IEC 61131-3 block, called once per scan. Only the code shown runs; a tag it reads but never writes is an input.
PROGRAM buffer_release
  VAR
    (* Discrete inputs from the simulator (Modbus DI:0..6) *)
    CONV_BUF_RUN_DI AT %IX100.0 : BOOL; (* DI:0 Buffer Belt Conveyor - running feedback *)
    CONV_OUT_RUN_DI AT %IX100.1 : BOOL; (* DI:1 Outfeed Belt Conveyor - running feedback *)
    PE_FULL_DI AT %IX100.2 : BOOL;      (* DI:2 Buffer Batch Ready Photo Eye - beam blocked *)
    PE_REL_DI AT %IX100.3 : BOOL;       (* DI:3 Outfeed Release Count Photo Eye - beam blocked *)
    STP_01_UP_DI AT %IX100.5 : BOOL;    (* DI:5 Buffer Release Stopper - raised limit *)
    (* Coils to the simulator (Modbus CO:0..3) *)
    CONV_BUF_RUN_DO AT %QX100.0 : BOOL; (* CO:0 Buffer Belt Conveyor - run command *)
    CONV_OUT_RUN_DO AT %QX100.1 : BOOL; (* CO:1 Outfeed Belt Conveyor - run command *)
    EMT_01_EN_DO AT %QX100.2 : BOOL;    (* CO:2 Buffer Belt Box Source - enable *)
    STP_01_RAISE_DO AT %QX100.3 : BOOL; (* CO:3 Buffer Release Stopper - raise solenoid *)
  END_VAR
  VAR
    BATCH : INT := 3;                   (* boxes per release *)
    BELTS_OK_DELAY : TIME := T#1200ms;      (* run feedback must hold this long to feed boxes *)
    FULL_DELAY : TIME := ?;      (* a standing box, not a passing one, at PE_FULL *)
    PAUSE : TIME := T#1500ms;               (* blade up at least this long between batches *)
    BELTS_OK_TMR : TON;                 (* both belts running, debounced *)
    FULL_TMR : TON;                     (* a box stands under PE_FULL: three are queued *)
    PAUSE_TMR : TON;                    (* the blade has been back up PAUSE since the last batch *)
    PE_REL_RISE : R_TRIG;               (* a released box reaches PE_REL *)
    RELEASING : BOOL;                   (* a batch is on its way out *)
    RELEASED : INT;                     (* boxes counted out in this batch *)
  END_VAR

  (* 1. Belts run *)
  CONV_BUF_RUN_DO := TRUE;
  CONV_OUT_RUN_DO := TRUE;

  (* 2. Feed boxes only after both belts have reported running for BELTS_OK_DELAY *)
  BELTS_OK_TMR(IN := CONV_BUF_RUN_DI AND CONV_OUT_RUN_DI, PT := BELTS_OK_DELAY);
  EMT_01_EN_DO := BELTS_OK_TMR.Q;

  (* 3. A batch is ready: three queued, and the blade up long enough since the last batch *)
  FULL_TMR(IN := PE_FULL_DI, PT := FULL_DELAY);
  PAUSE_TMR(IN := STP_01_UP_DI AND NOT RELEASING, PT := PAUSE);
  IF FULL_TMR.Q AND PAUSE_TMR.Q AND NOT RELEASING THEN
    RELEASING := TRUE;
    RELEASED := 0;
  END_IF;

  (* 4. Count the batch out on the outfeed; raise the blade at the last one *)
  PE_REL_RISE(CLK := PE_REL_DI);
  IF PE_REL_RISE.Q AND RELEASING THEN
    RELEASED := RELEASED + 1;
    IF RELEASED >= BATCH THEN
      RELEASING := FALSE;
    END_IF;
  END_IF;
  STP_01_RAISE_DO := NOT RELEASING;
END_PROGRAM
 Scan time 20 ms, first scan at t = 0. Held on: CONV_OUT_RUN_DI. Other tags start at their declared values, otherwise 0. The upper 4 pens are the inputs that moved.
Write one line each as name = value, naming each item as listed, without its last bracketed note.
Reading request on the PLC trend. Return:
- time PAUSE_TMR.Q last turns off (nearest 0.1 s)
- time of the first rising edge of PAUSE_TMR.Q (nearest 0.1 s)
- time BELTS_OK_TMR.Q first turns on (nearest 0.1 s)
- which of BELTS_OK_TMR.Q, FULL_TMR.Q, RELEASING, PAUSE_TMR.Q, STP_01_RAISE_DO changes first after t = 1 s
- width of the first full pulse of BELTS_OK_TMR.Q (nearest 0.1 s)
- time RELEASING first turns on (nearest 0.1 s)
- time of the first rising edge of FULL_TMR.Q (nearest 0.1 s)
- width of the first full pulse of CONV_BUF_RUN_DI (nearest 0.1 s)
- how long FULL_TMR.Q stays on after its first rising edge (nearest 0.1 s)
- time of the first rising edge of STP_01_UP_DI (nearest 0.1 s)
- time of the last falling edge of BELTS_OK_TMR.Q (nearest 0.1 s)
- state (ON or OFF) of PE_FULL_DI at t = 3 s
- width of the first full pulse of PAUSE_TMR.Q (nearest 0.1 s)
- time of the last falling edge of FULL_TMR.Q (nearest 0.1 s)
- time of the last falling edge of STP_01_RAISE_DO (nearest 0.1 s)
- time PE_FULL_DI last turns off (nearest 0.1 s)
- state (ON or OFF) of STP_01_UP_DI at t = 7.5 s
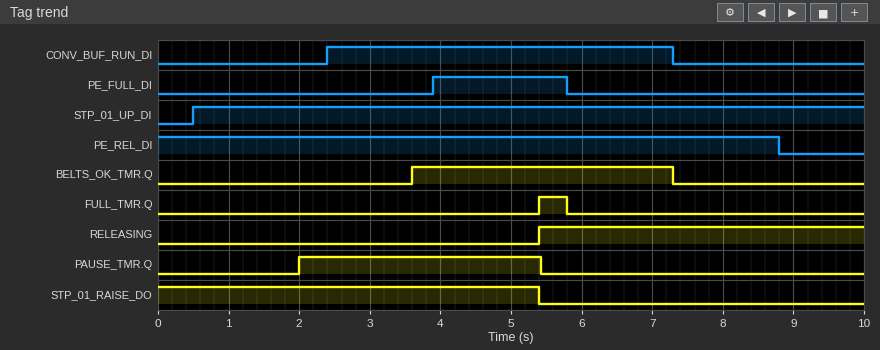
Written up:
time PAUSE_TMR.Q last turns off = 5.4 s
time of the first rising edge of PAUSE_TMR.Q = 2.0 s
time BELTS_OK_TMR.Q first turns on = 3.6 s
which of BELTS_OK_TMR.Q, FULL_TMR.Q, RELEASING, PAUSE_TMR.Q, STP_01_RAISE_DO changes first after t = 1 s = PAUSE_TMR.Q
width of the first full pulse of BELTS_OK_TMR.Q = 3.7 s
time RELEASING first turns on = 5.4 s
time of the first rising edge of FULL_TMR.Q = 5.4 s
width of the first full pulse of CONV_BUF_RUN_DI = 4.9 s
how long FULL_TMR.Q stays on after its first rising edge = 0.4 s
time of the first rising edge of STP_01_UP_DI = 0.5 s
time of the last falling edge of BELTS_OK_TMR.Q = 7.3 s
state (ON or OFF) of PE_FULL_DI at t = 3 s = OFF
width of the first full pulse of PAUSE_TMR.Q = 3.4 s
time of the last falling edge of FULL_TMR.Q = 5.8 s
time of the last falling edge of STP_01_RAISE_DO = 5.4 s
time PE_FULL_DI last turns off = 5.8 s
state (ON or OFF) of STP_01_UP_DI at t = 7.5 s = ON
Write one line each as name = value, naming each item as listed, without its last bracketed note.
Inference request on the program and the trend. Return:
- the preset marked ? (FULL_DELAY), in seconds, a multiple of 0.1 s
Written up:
the preset marked ? (FULL_DELAY), in seconds, a multiple of 0.1 s = 1.5 s
